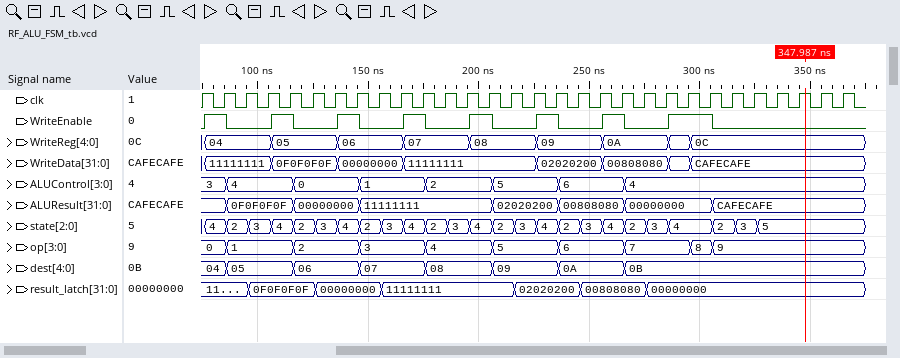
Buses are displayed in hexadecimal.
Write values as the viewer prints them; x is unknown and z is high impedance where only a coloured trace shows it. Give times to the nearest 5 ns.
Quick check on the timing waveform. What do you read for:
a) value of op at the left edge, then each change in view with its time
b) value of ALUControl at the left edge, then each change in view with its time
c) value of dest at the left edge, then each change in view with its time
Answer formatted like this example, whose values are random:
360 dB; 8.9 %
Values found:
0, 1 at 85 ns, 2 at 115 ns, 3 at 145 ns, 4 at 175 ns, 5 at 205 ns, 6 at 235 ns, 7 at 265 ns, 8 at 295 ns, 9 at 305 ns; 3, 4 at 85 ns, 0 at 115 ns, 1 at 145 ns, 2 at 175 ns, 5 at 205 ns, 6 at 235 ns, 4 at 265 ns; 04, 05 at 85 ns, 06 at 115 ns, 07 at 145 ns, 08 at 175 ns, 09 at 205 ns, 0A at 235 ns, 0B at 265 ns
